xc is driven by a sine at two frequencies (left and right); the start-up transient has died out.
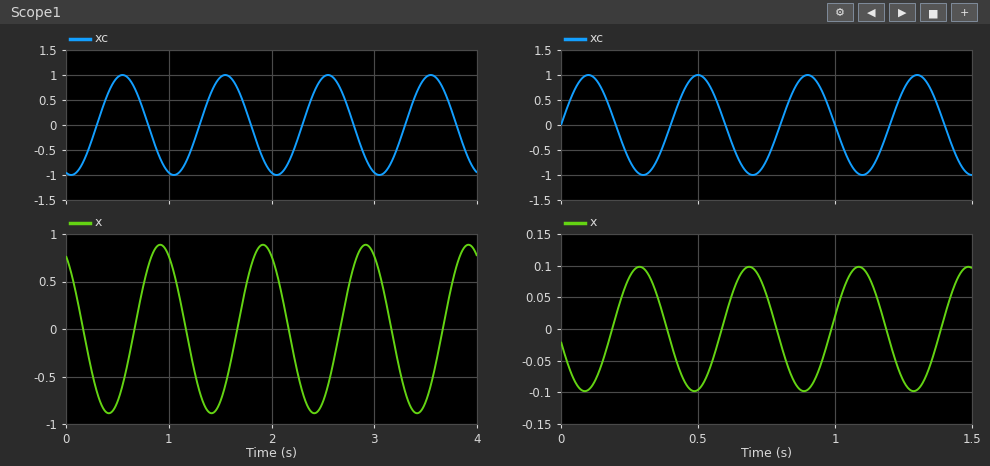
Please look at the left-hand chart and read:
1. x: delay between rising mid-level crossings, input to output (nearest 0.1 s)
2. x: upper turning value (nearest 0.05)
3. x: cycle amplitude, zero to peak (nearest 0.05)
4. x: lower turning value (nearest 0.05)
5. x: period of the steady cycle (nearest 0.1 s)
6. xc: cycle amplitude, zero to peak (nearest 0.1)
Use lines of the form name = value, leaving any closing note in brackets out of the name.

x: delay between rising mid-level crossings, input to output = 0.4 s
x: upper turning value = 0.90
x: cycle amplitude, zero to peak = 0.90
x: lower turning value = -0.90
x: period of the steady cycle = 1.0 s
xc: cycle amplitude, zero to peak = 1.0
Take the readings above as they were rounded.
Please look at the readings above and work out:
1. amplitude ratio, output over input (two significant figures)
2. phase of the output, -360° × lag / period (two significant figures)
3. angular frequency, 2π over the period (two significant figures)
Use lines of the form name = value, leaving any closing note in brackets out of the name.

amplitude ratio, output over input = 0.90
phase of the output, -360° × lag / period = -140°
angular frequency, 2π over the period = 6.3 rad/s
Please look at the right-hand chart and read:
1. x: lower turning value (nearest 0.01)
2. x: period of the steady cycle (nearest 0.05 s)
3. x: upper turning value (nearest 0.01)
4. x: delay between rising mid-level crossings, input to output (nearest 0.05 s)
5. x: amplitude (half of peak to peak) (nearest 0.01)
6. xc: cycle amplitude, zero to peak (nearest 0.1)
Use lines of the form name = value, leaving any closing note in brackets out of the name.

x: lower turning value = -0.10
x: period of the steady cycle = 0.40 s
x: upper turning value = 0.10
x: delay between rising mid-level crossings, input to output = 0.20 s
x: amplitude (half of peak to peak) = 0.10
xc: cycle amplitude, zero to peak = 1.0
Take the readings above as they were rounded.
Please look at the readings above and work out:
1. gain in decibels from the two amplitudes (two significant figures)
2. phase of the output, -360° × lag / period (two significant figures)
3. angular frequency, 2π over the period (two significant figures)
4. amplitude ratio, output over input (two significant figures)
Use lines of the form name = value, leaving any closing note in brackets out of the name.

gain in decibels from the two amplitudes = -20 dB
phase of the output, -360° × lag / period = -180°
angular frequency, 2π over the period = 16 rad/s
amplitude ratio, output over input = 0.10
